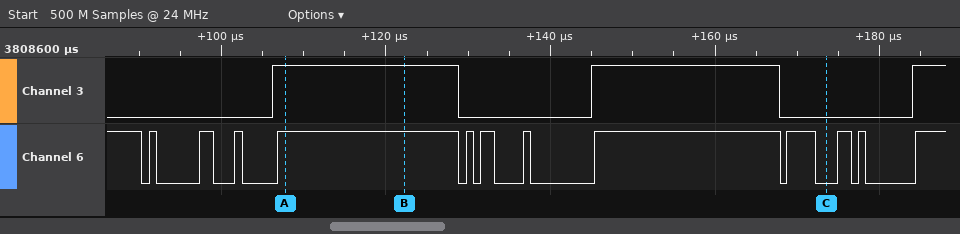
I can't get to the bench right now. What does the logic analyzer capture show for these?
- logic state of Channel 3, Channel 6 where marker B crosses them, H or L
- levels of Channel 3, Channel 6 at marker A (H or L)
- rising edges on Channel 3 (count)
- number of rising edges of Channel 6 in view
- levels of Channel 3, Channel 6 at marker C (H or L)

Channel 3=H, Channel 6=H
Channel 3=H, Channel 6=H
3
12
Channel 3=L, Channel 6=L
